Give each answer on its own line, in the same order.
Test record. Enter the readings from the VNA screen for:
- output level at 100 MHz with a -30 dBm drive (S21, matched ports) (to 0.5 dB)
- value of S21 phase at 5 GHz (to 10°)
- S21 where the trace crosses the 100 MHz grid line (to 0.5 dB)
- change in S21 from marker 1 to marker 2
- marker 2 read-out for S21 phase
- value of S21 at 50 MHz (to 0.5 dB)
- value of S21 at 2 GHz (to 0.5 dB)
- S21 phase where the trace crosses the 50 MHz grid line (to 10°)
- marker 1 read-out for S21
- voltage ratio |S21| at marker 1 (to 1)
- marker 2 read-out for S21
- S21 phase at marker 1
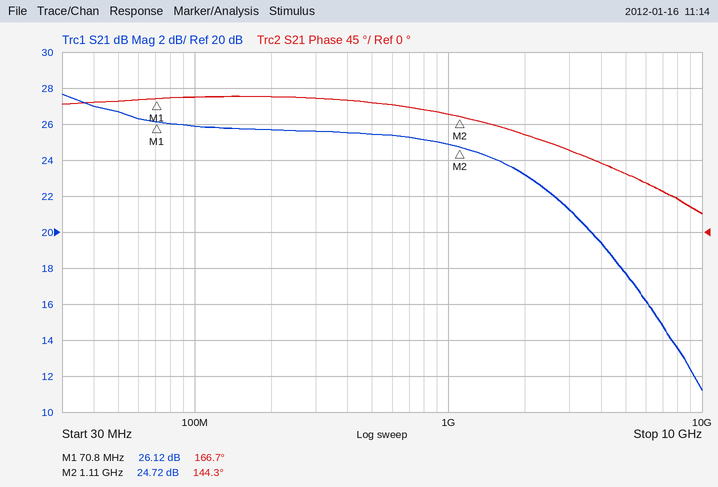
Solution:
-4.0 dBm
70°
26.0 dB
-1.40 dB
144.3°
26.5 dB
23.0 dB
160°
26.12 dB
20
24.72 dB
166.7°
